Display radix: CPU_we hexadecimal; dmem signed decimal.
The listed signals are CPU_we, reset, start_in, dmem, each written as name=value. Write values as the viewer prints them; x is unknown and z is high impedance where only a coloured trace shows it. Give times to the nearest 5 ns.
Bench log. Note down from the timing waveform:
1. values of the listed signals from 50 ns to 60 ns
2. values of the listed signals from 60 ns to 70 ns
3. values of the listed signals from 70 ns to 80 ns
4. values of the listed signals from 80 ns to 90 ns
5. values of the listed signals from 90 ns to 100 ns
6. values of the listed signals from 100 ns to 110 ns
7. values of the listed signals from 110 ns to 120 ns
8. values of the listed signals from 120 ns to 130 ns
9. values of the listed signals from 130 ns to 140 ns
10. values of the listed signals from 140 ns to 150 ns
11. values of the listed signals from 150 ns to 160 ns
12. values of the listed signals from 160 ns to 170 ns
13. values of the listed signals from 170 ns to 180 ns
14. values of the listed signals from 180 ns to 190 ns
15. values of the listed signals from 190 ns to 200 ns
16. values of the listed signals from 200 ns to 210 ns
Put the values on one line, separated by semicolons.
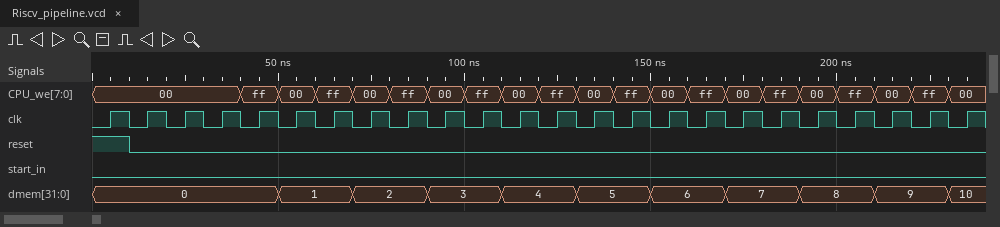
CPU_we=00, reset=0, start_in=0, dmem=1; CPU_we=ff, reset=0, start_in=0, dmem=1; CPU_we=00, reset=0, start_in=0, dmem=2; CPU_we=ff, reset=0, start_in=0, dmem=2; CPU_we=00, reset=0, start_in=0, dmem=3; CPU_we=ff, reset=0, start_in=0, dmem=3; CPU_we=00, reset=0, start_in=0, dmem=4; CPU_we=ff, reset=0, start_in=0, dmem=4; CPU_we=00, reset=0, start_in=0, dmem=5; CPU_we=ff, reset=0, start_in=0, dmem=5; CPU_we=00, reset=0, start_in=0, dmem=6; CPU_we=ff, reset=0, start_in=0, dmem=6; CPU_we=00, reset=0, start_in=0, dmem=7; CPU_we=ff, reset=0, start_in=0, dmem=7; CPU_we=00, reset=0, start_in=0, dmem=8; CPU_we=ff, reset=0, start_in=0, dmem=8
